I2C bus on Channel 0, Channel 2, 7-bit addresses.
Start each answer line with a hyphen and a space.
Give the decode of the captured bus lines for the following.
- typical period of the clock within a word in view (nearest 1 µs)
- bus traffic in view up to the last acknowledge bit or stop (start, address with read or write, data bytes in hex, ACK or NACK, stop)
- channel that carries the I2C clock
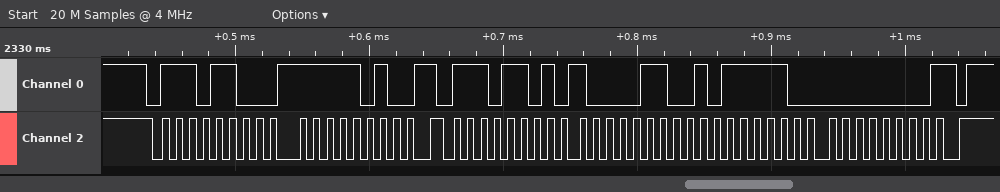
- 10 µs
- start, address 76 write ACK, FA ACK, repeated start, address 76 read ACK, 86 ACK, BE ACK, 00 NACK, stop
- Channel 2
